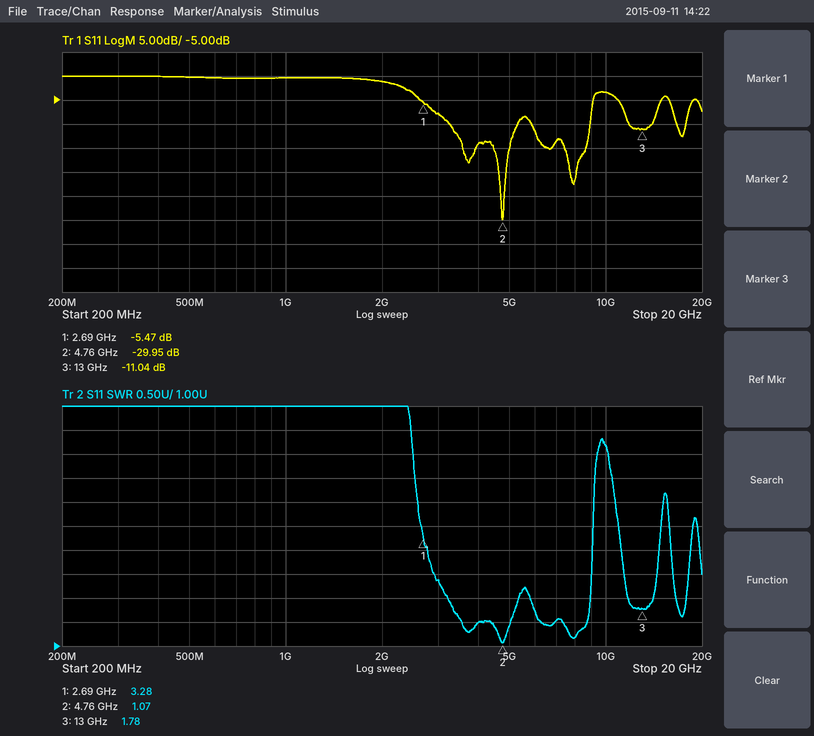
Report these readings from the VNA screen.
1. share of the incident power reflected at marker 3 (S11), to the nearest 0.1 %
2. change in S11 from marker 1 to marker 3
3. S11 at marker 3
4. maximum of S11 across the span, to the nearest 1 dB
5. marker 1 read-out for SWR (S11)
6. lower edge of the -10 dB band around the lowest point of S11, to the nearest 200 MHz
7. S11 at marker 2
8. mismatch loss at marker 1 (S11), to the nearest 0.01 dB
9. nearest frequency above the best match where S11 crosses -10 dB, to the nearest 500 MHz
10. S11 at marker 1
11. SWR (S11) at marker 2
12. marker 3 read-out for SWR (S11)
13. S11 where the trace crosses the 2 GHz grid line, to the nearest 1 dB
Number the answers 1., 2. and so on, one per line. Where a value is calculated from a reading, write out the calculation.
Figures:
1. 10^(-11.04/10) ≈ 7.9 %
2. -11.04 − (-5.47) = -5.57 dB
3. -11.04 dB
4. 0 dB
5. 3.28
6. 3.2 GHz
7. -29.95 dB
8. −10 log10(1 − 10^(-5.47/10)) ≈ 1.45 dB
9. 5.5 GHz
10. -5.47 dB
11. 1.07
12. 1.78
13. -1 dB
